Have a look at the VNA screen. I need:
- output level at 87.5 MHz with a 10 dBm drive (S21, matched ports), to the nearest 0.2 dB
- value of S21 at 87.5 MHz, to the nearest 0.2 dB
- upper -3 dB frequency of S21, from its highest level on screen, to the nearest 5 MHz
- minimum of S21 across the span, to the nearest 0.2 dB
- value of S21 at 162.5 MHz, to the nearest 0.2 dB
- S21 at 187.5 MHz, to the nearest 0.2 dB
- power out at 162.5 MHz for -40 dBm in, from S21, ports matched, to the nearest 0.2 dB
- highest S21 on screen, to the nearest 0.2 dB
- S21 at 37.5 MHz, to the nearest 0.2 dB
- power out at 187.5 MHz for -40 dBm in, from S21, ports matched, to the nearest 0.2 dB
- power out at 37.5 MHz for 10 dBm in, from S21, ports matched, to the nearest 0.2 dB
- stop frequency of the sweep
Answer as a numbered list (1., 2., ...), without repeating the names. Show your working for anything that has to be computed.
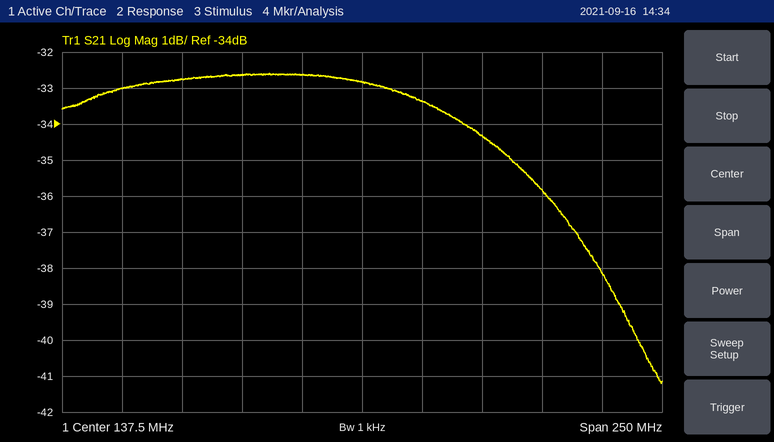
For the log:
1. 10 dBm + (-32.6 dB) = -22.6 dBm
2. -32.6 dB
3. 210 MHz
4. -41.2 dB
5. -33.4 dB
6. -34.4 dB
7. -40 dBm + (-33.4 dB) = -73.4 dBm
8. -32.6 dB
9. -33.0 dB
10. -40 dBm + (-34.4 dB) = -74.4 dBm
11. 10 dBm + (-33.0 dB) = -23.0 dBm
12. 262.5 MHz
